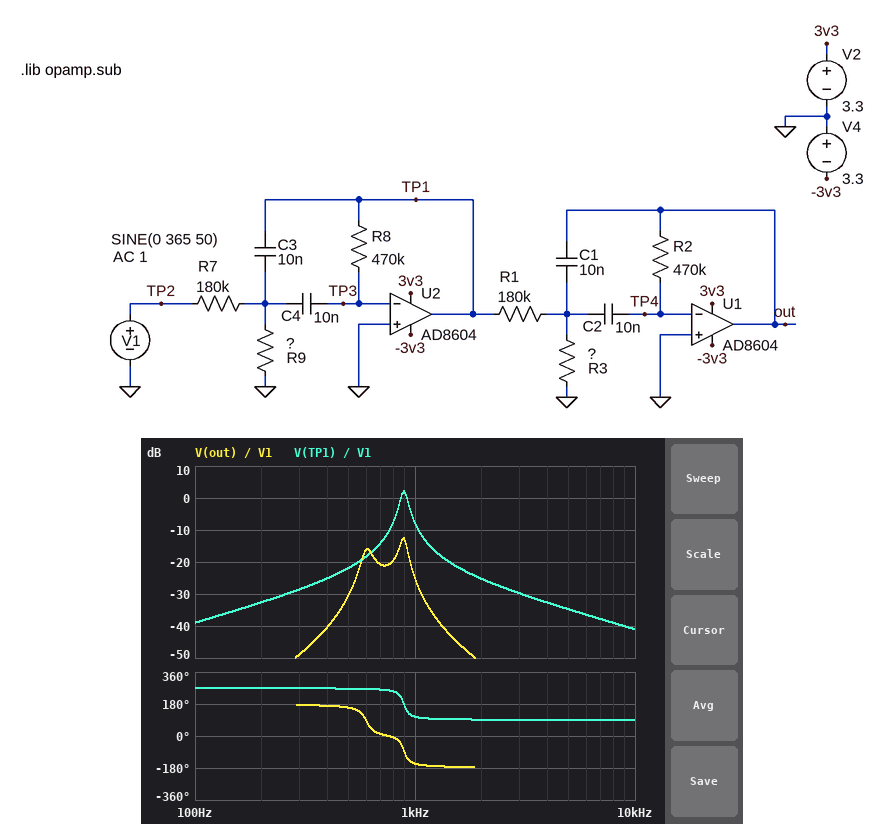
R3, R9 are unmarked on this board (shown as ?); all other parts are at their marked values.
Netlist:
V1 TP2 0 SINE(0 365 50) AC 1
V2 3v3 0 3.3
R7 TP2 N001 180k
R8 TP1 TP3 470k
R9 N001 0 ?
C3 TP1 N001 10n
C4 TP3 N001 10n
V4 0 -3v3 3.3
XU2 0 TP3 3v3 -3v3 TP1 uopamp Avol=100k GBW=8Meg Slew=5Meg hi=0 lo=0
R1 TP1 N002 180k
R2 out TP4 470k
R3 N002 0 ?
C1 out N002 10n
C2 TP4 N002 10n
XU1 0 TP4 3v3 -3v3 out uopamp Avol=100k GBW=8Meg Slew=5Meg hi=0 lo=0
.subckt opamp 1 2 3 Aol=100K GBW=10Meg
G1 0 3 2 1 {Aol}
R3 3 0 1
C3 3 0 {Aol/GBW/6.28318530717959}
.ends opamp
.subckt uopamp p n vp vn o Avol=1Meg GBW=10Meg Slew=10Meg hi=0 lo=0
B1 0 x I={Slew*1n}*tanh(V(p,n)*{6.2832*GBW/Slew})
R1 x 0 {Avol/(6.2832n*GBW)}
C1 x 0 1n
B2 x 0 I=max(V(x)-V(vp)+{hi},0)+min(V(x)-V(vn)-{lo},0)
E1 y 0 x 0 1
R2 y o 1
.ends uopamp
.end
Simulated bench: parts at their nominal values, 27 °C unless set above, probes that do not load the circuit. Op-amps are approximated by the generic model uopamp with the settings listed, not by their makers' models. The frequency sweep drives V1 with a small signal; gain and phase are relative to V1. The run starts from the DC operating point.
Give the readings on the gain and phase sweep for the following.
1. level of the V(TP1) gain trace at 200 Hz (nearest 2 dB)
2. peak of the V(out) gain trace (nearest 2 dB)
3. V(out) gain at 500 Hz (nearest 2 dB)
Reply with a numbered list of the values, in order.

1. -32 dB
2. -12 dB
3. -30 dB
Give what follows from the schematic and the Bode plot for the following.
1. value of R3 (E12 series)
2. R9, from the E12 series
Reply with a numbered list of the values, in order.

1. 1.5 kΩ
2. 680 Ω
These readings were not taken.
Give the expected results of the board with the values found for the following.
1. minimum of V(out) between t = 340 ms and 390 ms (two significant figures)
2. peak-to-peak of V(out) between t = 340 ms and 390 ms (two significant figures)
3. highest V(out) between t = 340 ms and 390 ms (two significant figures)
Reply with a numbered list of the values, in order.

1. -25 mV
2. 50 mV
3. 25 mV
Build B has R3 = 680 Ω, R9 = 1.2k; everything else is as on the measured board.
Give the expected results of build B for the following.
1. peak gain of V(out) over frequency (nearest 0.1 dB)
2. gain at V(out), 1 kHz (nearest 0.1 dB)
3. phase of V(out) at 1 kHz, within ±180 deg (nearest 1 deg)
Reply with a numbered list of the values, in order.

1. -10.5 dB
2. -23.8 dB
3. -155 deg
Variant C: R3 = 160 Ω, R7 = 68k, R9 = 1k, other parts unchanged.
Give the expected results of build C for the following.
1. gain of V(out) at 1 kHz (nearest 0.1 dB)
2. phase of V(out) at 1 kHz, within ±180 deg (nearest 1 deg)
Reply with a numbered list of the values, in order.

1. -34.4 dB
2. 7 deg
